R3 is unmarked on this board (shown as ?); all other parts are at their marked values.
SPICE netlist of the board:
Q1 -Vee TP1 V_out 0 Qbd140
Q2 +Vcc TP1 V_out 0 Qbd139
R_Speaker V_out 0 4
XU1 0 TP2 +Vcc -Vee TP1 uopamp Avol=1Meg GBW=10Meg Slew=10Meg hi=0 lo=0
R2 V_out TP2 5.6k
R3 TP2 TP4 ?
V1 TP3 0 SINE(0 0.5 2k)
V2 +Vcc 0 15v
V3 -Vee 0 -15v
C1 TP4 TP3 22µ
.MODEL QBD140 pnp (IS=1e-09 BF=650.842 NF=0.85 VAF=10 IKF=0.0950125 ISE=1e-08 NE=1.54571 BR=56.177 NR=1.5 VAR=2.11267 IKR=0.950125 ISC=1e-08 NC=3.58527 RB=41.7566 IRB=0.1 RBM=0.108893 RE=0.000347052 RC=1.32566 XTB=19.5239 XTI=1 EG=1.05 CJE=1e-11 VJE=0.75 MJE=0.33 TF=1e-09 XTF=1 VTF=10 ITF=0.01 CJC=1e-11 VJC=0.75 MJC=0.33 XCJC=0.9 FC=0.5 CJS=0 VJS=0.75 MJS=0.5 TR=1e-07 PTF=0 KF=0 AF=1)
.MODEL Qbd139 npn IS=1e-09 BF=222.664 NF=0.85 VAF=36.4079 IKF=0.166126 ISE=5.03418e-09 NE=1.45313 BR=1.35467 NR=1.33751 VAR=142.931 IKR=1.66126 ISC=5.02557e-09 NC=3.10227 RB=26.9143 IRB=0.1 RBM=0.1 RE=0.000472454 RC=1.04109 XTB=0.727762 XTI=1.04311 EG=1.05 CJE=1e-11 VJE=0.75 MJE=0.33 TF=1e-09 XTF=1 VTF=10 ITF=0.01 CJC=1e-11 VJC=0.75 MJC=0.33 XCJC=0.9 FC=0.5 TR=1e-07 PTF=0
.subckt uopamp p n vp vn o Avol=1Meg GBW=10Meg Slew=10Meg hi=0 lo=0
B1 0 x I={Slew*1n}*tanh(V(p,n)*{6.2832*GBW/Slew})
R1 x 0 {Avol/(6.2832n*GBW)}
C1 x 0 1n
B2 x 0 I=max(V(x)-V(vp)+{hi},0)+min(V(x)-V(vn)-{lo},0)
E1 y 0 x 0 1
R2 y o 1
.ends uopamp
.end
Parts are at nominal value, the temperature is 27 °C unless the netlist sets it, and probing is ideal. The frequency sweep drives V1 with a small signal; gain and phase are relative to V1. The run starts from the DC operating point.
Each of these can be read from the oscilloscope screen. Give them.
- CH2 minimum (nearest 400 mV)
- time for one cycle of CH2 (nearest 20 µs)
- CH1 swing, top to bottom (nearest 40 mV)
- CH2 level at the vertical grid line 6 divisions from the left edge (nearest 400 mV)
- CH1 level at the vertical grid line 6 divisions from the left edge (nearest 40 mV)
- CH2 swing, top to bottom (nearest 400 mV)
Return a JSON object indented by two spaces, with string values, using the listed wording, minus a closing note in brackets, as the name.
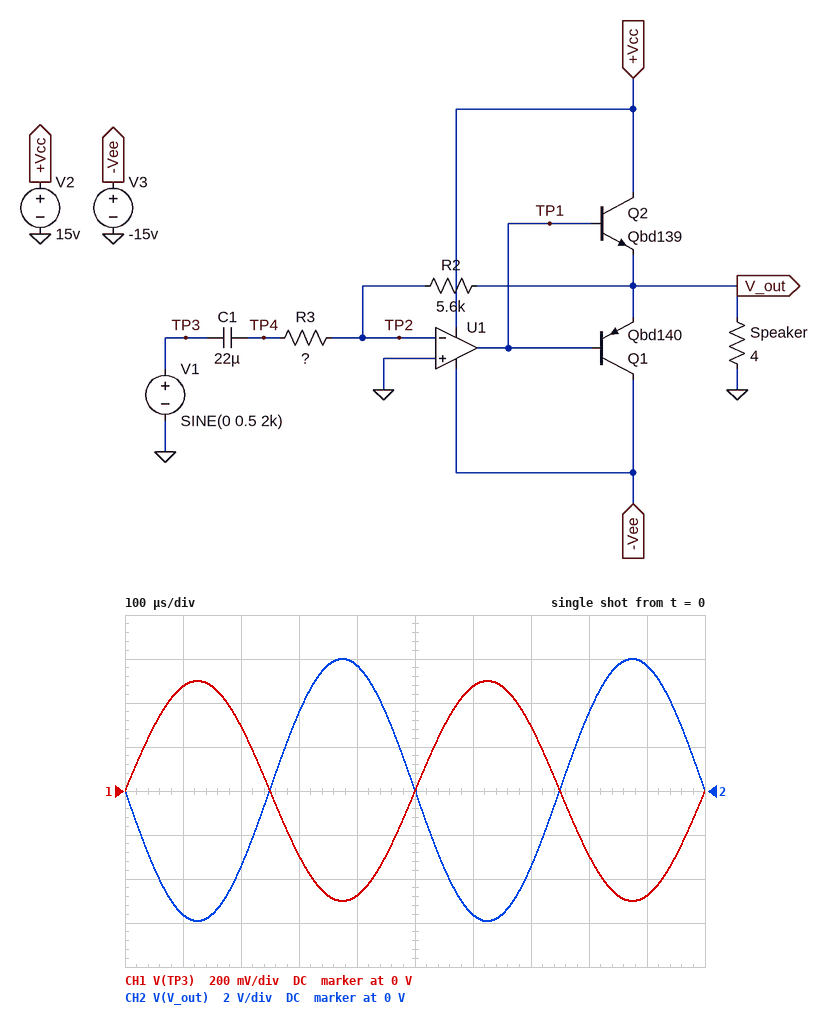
{
  "CH2 minimum": "-6.0 V",
  "time for one cycle of CH2": "500 µs",
  "CH1 swing, top to bottom": "1.00 V",
  "CH2 level at the vertical grid line 6 divisions from the left edge": "-5.6 V",
  "CH1 level at the vertical grid line 6 divisions from the left edge": "480 mV",
  "CH2 swing, top to bottom": "12.0 V"
}
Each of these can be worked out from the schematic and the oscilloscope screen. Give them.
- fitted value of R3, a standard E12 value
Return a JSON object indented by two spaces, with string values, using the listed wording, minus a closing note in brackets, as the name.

{
  "fitted value of R3, a standard E12 value": "470 Ω"
}
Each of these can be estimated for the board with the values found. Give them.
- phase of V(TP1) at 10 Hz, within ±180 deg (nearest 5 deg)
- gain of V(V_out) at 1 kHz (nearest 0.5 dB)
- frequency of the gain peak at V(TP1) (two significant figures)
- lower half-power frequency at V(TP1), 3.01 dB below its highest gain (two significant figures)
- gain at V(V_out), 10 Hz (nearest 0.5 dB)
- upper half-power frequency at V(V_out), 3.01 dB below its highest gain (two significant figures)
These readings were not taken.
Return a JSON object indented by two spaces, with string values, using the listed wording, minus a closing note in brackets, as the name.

{
  "phase of V(TP1) at 10 Hz, within ±180 deg": "155 deg",
  "gain of V(V_out) at 1 kHz": "-33.5 dB",
  "frequency of the gain peak at V(TP1)": "6.2 Hz",
  "lower half-power frequency at V(TP1), 3.01 dB below its highest gain": "2.5 Hz",
  "gain at V(V_out), 10 Hz": "3.0 dB",
  "upper half-power frequency at V(V_out), 3.01 dB below its highest gain": "15 Hz"
}
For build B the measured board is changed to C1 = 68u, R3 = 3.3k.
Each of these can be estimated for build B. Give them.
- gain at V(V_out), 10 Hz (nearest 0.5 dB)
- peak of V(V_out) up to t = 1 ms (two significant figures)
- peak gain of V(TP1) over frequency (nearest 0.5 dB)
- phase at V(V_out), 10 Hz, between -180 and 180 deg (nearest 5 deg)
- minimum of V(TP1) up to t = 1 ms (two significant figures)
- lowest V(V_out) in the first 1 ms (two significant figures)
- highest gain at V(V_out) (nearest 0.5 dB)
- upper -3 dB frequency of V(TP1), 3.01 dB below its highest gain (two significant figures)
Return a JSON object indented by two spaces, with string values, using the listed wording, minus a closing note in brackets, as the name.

{
  "gain at V(V_out), 10 Hz": "-3.5 dB",
  "peak of V(V_out) up to t = 1 ms": "850 mV",
  "peak gain of V(TP1) over frequency": "110.5 dB",
  "phase at V(V_out), 10 Hz, between -180 and 180 deg": "155 deg",
  "minimum of V(TP1) up to t = 1 ms": "-1.3 V",
  "lowest V(V_out) in the first 1 ms": "-850 mV",
  "highest gain at V(V_out)": "-2.5 dB",
  "upper -3 dB frequency of V(TP1), 3.01 dB below its highest gain": "19 Hz"
}
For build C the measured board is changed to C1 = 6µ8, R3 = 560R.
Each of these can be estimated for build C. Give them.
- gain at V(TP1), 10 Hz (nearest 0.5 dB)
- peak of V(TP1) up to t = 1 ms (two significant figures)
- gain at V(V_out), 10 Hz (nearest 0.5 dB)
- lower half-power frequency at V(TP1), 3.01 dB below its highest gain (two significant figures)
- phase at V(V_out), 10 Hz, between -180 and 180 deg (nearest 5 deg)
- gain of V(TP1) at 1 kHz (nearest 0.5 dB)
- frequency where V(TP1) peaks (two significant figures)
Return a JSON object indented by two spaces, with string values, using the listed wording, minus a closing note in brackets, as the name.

{
  "gain at V(TP1), 10 Hz": "115.0 dB",
  "peak of V(TP1) up to t = 1 ms": "6.2 V",
  "gain at V(V_out), 10 Hz": "2.0 dB",
  "lower half-power frequency at V(TP1), 3.01 dB below its highest gain": "5.7 Hz",
  "phase at V(V_out), 10 Hz, between -180 and 180 deg": "-170 deg",
  "gain of V(TP1) at 1 kHz": "79.0 dB",
  "frequency where V(TP1) peaks": "11 Hz"
}
